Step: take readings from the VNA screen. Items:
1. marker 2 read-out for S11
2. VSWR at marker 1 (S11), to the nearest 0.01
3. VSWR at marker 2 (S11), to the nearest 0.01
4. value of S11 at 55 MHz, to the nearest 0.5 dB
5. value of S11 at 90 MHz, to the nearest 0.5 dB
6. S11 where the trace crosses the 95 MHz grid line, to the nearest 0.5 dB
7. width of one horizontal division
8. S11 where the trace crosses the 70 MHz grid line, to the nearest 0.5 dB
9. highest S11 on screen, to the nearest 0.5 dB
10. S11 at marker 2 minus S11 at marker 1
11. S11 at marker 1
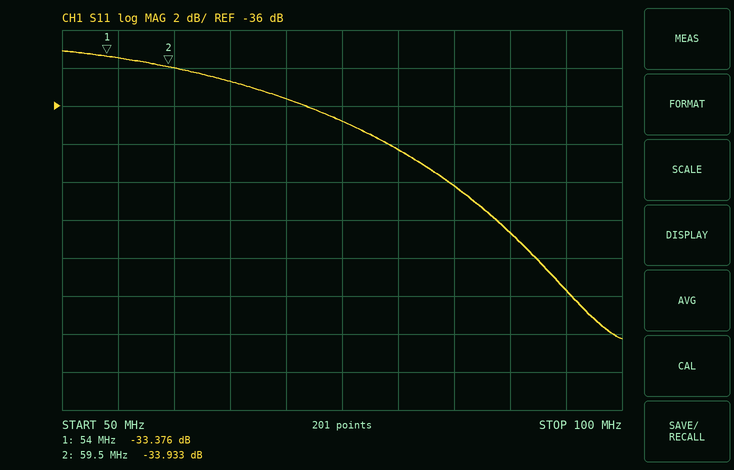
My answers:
-33.933 dB
1.04
1.04
-33.5 dB
-42.5 dB
-45.5 dB
5 MHz
-35.5 dB
-33.0 dB
-0.557 dB
-33.376 dB
